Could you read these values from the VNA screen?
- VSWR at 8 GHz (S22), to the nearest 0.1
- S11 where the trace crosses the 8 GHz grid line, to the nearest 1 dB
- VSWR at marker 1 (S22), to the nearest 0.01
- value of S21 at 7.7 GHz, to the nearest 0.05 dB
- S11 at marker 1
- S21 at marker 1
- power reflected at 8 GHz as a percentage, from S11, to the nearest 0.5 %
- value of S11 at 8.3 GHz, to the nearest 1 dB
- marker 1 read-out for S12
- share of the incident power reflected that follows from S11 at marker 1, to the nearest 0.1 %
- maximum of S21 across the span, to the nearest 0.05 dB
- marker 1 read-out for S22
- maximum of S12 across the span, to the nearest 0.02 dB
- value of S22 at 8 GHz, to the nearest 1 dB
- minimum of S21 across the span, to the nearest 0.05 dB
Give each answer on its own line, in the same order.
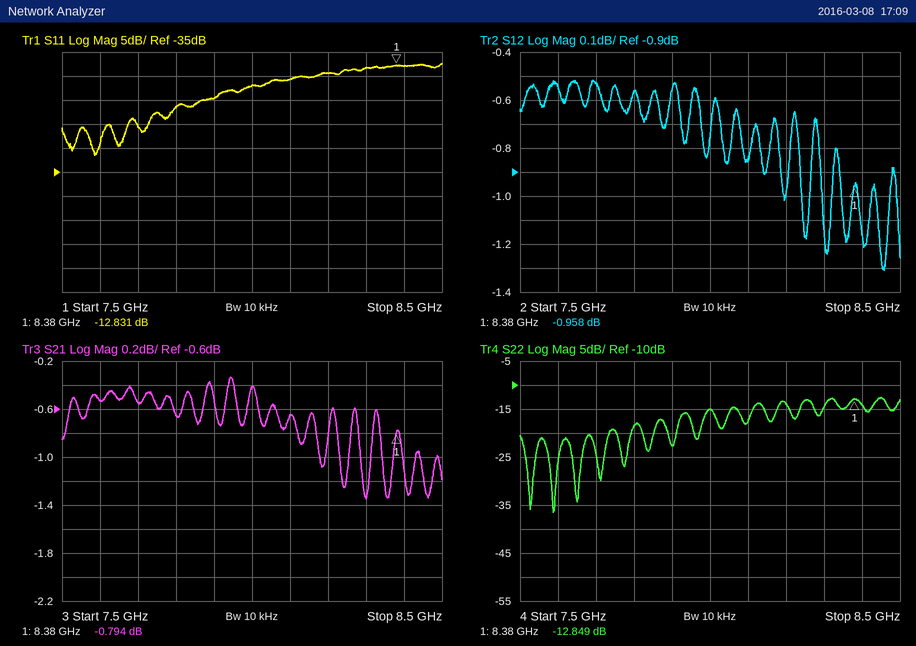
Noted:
1.4
-17 dB
1.59
-0.55 dB
-12.831 dB
-0.794 dB
2.0 %
-13 dB
-0.958 dB
5.2 %
-0.35 dB
-12.849 dB
-0.52 dB
-15 dB
-1.35 dB
